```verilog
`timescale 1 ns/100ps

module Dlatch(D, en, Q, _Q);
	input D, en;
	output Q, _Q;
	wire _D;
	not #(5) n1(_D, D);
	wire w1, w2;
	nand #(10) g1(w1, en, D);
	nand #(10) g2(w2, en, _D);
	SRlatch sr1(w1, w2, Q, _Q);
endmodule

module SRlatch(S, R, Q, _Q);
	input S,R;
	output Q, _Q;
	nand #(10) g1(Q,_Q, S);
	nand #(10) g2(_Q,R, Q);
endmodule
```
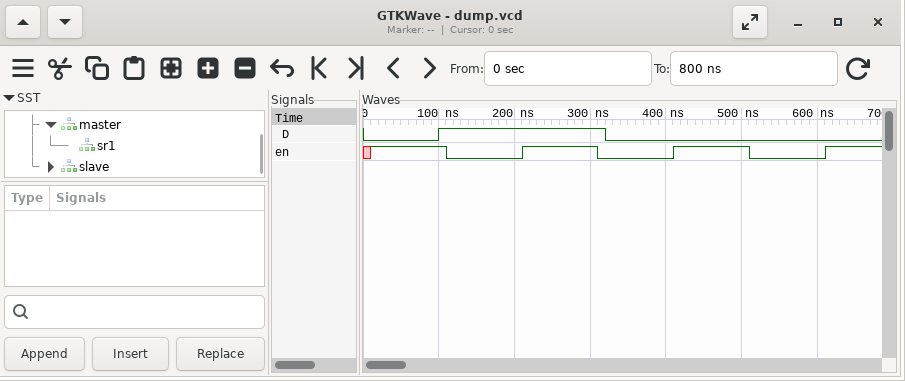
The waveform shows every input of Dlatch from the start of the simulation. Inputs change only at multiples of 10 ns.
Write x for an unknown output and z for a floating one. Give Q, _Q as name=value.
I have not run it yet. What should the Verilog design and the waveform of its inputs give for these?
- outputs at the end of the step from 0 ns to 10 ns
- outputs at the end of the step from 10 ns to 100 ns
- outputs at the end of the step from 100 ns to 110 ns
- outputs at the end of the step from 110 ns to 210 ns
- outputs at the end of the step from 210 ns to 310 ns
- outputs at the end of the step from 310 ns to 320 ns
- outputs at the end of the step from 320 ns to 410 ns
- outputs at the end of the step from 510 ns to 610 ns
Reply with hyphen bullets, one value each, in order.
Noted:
- Q=x, _Q=x
- Q=0, _Q=1
- Q=0, _Q=1
- Q=1, _Q=1
- Q=1, _Q=0
- Q=1, _Q=0
- Q=1, _Q=0
- Q=0, _Q=1
